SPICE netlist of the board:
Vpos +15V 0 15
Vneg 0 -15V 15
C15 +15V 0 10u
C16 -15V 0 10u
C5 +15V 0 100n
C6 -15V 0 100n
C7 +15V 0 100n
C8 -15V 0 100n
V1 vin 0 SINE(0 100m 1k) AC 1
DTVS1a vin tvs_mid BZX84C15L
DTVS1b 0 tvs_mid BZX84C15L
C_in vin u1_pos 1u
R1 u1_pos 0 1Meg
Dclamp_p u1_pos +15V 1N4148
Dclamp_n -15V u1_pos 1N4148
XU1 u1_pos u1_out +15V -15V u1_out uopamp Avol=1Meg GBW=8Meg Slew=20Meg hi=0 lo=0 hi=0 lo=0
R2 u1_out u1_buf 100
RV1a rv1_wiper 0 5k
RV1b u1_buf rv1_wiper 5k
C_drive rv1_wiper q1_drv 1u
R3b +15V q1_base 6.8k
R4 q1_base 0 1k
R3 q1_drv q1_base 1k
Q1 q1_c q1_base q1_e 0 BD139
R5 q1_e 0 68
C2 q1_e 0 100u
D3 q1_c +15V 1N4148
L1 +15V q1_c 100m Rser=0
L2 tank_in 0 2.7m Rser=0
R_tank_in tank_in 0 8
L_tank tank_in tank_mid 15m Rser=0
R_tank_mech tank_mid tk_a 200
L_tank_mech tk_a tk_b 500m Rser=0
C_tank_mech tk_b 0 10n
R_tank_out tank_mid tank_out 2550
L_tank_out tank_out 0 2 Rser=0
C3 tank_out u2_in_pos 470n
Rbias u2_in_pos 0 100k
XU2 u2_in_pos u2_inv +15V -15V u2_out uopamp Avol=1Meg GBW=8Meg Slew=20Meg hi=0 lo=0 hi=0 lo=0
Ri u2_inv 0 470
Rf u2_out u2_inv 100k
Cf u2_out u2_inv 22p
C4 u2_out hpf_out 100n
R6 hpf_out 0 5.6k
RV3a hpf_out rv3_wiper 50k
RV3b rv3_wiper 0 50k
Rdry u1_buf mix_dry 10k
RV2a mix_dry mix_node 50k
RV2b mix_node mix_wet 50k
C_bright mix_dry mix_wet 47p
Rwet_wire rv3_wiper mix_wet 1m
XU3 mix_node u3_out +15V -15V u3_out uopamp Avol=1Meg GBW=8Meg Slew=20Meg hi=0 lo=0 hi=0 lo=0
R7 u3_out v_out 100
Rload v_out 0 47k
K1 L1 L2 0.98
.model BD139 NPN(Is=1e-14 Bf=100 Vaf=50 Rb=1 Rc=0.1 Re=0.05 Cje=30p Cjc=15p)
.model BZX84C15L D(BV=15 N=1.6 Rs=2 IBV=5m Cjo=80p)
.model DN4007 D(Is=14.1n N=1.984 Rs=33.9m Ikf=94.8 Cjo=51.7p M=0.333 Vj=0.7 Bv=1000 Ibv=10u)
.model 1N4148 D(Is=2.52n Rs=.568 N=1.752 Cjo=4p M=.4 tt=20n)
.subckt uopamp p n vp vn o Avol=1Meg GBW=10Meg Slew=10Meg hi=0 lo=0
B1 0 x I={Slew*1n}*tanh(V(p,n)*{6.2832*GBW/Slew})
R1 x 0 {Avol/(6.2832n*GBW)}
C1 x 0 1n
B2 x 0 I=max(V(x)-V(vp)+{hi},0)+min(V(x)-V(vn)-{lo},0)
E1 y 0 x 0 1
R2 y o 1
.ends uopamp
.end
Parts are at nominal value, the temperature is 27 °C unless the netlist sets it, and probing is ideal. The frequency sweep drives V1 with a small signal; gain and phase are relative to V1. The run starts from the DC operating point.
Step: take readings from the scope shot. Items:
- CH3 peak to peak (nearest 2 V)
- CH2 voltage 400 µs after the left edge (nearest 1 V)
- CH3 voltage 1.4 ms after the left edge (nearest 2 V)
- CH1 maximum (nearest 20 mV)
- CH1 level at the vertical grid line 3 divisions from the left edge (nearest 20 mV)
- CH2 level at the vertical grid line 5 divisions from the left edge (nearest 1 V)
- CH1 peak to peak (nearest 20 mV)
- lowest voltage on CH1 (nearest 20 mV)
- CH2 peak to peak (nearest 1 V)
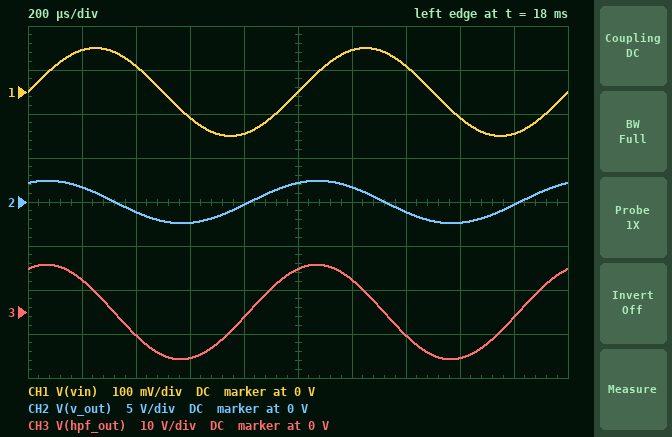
22 V
-1 V
-6 V
100 mV
-60 mV
2 V
200 mV
-100 mV
5 V
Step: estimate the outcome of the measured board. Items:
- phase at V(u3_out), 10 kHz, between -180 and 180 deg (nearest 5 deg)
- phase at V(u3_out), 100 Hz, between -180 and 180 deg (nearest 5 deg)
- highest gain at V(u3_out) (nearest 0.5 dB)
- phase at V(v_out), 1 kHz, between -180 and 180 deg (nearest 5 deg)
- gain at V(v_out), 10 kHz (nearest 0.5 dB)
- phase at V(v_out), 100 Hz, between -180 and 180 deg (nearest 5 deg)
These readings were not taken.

-20 deg
-25 deg
33.5 dB
65 deg
28.5 dB
-25 deg
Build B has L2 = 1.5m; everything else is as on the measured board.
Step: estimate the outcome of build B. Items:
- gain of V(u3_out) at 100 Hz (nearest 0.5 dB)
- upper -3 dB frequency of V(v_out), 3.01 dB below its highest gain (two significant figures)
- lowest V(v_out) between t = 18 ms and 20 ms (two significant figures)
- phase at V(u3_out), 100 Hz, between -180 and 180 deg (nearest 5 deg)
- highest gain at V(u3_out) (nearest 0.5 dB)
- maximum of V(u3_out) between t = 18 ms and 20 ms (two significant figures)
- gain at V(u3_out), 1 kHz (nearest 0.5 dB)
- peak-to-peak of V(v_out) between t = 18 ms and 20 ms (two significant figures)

-3.5 dB
2.2 kHz
-2.6 V
-20 deg
35.5 dB
2.7 V
28.5 dB
5.2 V
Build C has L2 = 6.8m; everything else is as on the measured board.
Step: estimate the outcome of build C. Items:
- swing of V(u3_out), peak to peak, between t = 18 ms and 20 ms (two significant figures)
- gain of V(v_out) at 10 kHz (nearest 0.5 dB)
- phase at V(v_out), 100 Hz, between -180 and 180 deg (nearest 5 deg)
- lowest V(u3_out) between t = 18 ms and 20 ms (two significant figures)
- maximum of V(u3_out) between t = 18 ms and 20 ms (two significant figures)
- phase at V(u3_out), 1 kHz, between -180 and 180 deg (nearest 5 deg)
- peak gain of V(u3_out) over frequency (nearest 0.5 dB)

3.4 V
25.0 dB
-40 deg
-1.7 V
1.7 V
50 deg
29.5 dB
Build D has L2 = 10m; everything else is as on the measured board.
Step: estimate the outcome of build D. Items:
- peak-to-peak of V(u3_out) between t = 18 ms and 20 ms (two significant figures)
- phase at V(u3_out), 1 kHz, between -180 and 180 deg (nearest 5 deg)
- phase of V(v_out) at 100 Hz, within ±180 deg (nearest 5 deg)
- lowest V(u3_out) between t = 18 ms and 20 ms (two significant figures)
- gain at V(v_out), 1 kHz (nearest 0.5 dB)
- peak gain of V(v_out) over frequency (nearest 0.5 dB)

2.9 V
45 deg
-45 deg
-1.4 V
23.0 dB
28.0 dB
